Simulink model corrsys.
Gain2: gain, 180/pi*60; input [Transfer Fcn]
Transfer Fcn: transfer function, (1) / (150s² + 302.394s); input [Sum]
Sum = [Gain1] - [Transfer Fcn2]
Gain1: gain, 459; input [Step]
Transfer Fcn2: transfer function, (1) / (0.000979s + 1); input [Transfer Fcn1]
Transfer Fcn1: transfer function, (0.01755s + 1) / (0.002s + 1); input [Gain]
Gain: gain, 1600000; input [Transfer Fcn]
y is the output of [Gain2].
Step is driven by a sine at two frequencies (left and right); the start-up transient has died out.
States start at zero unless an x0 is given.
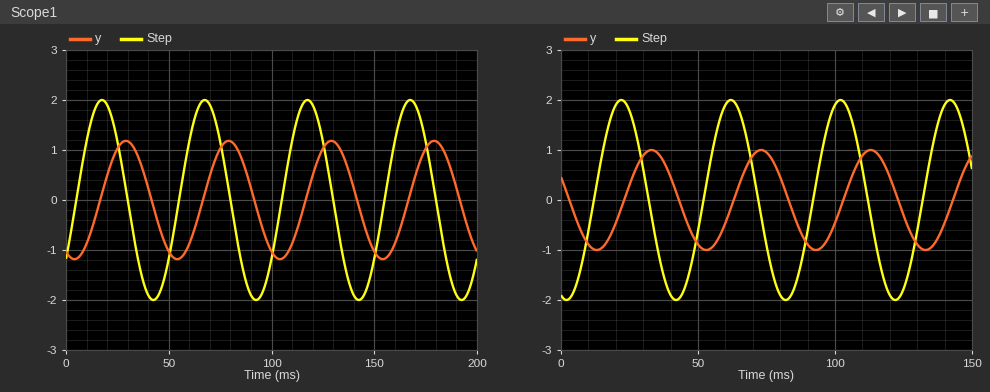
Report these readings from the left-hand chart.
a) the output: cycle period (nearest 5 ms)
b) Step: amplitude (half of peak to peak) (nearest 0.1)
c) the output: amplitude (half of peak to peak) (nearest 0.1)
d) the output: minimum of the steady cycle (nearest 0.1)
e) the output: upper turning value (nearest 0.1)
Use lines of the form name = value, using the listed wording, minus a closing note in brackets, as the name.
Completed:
the output: cycle period = 50 ms
Step: amplitude (half of peak to peak) = 2.0
the output: amplitude (half of peak to peak) = 1.2
the output: minimum of the steady cycle = -1.2
the output: upper turning value = 1.2
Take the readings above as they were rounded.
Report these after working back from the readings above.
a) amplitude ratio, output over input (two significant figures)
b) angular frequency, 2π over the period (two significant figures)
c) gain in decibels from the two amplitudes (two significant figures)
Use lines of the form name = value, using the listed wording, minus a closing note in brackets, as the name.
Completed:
amplitude ratio, output over input = 0.60
angular frequency, 2π over the period = 0.13 rad/ms
gain in decibels from the two amplitudes = -4.4 dB
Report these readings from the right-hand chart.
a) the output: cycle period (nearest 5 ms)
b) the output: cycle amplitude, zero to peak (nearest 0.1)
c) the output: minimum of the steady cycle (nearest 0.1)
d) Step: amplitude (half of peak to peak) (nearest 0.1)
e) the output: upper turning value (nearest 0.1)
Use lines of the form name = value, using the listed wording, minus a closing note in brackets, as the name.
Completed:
the output: cycle period = 40 ms
the output: cycle amplitude, zero to peak = 1.0
the output: minimum of the steady cycle = -1.0
Step: amplitude (half of peak to peak) = 2.0
the output: upper turning value = 1.0
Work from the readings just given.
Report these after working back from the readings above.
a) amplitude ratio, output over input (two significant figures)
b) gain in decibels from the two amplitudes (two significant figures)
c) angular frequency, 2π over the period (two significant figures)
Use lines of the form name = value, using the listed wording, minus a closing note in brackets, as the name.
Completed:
amplitude ratio, output over input = 0.50
gain in decibels from the two amplitudes = -6.0 dB
angular frequency, 2π over the period = 0.16 rad/ms
